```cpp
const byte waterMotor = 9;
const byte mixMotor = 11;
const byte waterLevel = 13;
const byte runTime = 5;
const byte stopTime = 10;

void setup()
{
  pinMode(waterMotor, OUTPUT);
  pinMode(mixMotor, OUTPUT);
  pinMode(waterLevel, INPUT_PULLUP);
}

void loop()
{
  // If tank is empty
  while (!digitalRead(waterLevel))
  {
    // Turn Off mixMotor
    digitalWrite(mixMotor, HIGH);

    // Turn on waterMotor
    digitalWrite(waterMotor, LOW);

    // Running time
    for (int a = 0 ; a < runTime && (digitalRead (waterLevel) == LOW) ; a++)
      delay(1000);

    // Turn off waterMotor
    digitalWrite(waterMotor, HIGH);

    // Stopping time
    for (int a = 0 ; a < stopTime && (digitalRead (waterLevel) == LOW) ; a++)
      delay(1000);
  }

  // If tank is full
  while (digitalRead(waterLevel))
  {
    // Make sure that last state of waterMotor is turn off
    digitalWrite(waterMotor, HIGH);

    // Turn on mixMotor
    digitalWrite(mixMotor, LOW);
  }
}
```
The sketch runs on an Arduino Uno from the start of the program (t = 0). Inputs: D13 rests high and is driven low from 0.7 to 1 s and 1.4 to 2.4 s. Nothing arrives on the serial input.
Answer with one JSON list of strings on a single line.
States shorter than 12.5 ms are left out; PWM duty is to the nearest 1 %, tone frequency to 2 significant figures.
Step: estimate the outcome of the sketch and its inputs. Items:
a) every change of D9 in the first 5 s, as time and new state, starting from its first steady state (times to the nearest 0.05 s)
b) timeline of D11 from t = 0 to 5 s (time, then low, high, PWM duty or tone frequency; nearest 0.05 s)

["0 s high; 0.7 s low; 2.7 s high", "0 s low; 0.7 s high; 2.7 s low"]
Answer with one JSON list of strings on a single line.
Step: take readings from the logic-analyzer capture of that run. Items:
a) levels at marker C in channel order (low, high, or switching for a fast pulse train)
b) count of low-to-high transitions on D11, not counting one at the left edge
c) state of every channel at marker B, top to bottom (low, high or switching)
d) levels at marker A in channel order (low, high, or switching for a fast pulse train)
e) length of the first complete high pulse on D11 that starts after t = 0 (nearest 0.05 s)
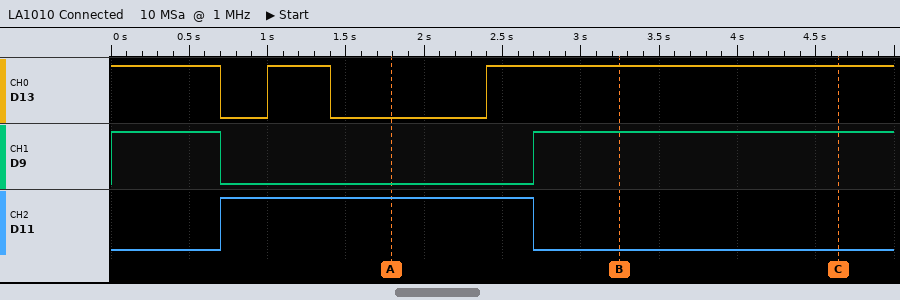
["D13 high, D9 high, D11 low", "1", "D13 high, D9 high, D11 low", "D13 low, D9 low, D11 high", "2.00 s"]
